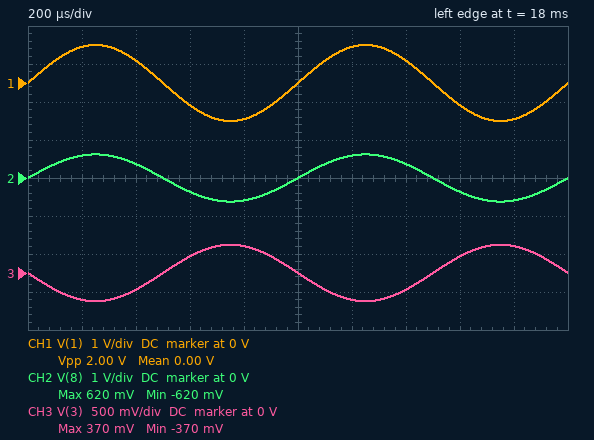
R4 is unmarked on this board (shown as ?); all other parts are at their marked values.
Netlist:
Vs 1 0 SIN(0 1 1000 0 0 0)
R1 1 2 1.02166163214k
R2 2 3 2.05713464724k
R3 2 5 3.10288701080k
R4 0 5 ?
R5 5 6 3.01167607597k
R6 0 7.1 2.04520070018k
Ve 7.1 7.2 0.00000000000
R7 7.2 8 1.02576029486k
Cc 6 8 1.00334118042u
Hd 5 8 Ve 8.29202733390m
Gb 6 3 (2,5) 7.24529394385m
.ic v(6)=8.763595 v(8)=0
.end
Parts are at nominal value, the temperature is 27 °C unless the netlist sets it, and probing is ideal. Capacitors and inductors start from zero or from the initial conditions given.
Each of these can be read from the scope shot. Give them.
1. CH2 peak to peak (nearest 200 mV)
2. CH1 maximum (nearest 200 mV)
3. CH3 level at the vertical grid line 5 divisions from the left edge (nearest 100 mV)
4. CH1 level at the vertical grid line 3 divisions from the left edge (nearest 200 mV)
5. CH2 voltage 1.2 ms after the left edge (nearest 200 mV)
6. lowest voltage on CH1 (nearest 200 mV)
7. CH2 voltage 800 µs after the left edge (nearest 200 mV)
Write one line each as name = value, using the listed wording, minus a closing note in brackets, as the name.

CH2 peak to peak = 1.2 V
CH1 maximum = 1.0 V
CH3 level at the vertical grid line 5 divisions from the left edge = 0 V
CH1 level at the vertical grid line 3 divisions from the left edge = -600 mV
CH2 voltage 1.2 ms after the left edge = 600 mV
lowest voltage on CH1 = -1.0 V
CH2 voltage 800 µs after the left edge = -600 mV
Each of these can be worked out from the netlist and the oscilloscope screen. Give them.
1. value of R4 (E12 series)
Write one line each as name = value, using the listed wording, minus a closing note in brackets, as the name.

value of R4 = 2.7 kΩ
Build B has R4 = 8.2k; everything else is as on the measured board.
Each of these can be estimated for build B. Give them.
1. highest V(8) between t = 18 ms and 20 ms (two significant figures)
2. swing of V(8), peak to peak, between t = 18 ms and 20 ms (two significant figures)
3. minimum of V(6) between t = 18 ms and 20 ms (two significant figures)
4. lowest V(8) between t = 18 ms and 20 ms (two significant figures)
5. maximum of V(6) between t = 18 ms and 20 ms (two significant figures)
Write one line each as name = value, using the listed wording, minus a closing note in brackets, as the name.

highest V(8) between t = 18 ms and 20 ms = 720 mV
swing of V(8), peak to peak, between t = 18 ms and 20 ms = 1.4 V
minimum of V(6) between t = 18 ms and 20 ms = -710 mV
lowest V(8) between t = 18 ms and 20 ms = -720 mV
maximum of V(6) between t = 18 ms and 20 ms = 740 mV
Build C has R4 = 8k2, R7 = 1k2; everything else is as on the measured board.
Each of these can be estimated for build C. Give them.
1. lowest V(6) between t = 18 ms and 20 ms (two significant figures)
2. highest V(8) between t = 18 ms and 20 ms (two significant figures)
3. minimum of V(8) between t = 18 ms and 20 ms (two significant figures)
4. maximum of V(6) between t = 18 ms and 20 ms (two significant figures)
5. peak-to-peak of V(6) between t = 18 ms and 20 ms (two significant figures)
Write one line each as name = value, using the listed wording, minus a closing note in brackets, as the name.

lowest V(6) between t = 18 ms and 20 ms = -720 mV
highest V(8) between t = 18 ms and 20 ms = 730 mV
minimum of V(8) between t = 18 ms and 20 ms = -730 mV
maximum of V(6) between t = 18 ms and 20 ms = 750 mV
peak-to-peak of V(6) between t = 18 ms and 20 ms = 1.5 V
